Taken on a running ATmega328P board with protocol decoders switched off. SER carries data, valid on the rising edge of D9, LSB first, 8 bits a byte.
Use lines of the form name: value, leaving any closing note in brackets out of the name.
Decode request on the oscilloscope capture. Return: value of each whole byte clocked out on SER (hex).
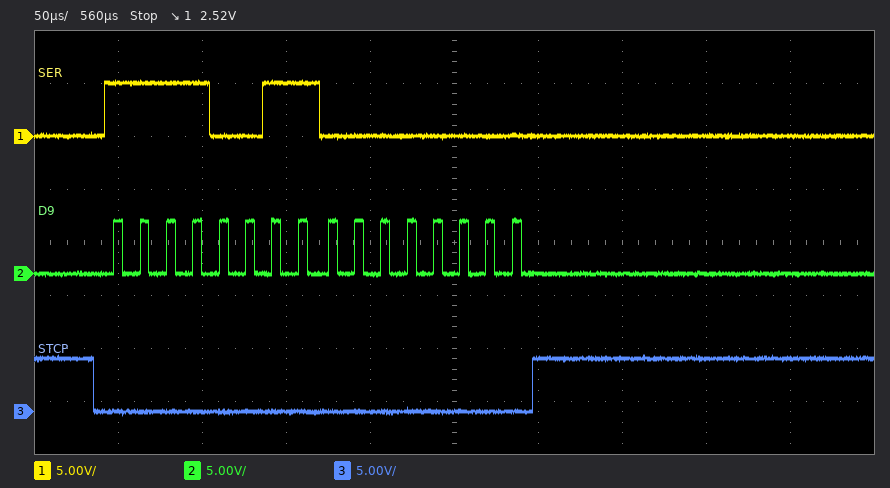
value of each whole byte clocked out on SER: 0xCF 0x00
